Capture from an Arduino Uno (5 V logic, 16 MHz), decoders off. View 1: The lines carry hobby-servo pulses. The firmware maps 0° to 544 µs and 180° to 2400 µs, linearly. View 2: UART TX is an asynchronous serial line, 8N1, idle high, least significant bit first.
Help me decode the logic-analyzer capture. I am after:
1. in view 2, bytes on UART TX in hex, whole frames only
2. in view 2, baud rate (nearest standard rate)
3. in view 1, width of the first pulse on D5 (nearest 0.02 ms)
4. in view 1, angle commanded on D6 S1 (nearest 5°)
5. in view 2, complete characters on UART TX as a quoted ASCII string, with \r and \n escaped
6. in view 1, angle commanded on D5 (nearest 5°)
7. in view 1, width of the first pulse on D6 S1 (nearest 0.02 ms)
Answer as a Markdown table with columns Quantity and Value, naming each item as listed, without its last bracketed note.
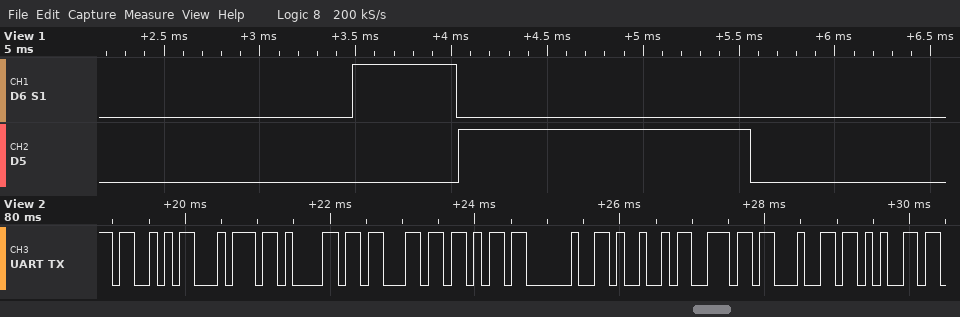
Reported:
| Quantity | Value |
|---|---|
| in view 2, bytes on UART TX in hex, whole frames only | 53 74 61 63 6B 20 49 6E 64 65 |
| in view 2, baud rate | 9600 baud |
| in view 1, width of the first pulse on D5 | 1.52 ms |
| in view 1, angle commanded on D6 S1 | 0° |
| in view 2, complete characters on UART TX as a quoted ASCII string, with \r and \n escaped | "Stack Inde" |
| in view 1, angle commanded on D5 | 95° |
| in view 1, width of the first pulse on D6 S1 | 0.54 ms |
